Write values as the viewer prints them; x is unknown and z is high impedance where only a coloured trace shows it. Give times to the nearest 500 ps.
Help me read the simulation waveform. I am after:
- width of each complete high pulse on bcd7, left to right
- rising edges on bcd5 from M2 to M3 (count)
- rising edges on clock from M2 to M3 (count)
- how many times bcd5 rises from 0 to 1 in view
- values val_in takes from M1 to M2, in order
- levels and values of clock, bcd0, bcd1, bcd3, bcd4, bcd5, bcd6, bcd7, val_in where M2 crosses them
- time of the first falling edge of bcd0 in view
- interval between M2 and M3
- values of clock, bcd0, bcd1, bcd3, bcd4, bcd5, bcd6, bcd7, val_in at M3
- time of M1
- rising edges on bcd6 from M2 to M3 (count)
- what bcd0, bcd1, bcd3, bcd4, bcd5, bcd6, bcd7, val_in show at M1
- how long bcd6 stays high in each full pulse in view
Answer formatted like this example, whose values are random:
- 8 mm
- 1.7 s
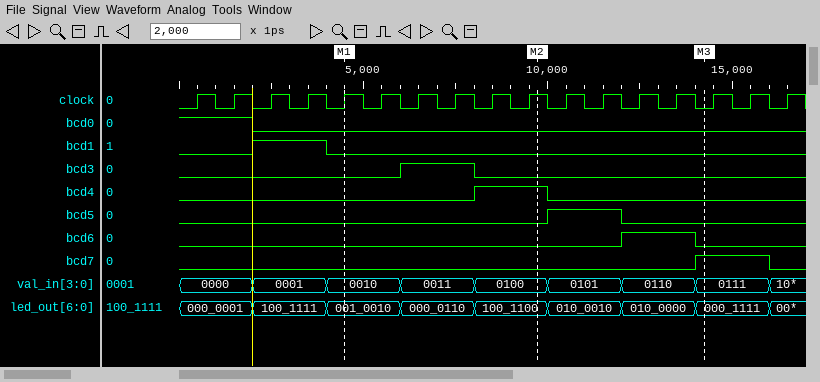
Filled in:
- 2000 ps
- 1
- 4
- 1
- 0010, 0011, 0100
- clock=1, bcd0=0, bcd1=0, bcd3=0, bcd4=1, bcd5=0, bcd6=0, bcd7=0, val_in=0100
- 2000 ps
- 4500 ps
- clock=0, bcd0=0, bcd1=0, bcd3=0, bcd4=0, bcd5=0, bcd6=0, bcd7=1, val_in=0111
- 4500 ps
- 1
- bcd0=0, bcd1=0, bcd3=0, bcd4=0, bcd5=0, bcd6=0, bcd7=0, val_in=0010
- 2000 ps
